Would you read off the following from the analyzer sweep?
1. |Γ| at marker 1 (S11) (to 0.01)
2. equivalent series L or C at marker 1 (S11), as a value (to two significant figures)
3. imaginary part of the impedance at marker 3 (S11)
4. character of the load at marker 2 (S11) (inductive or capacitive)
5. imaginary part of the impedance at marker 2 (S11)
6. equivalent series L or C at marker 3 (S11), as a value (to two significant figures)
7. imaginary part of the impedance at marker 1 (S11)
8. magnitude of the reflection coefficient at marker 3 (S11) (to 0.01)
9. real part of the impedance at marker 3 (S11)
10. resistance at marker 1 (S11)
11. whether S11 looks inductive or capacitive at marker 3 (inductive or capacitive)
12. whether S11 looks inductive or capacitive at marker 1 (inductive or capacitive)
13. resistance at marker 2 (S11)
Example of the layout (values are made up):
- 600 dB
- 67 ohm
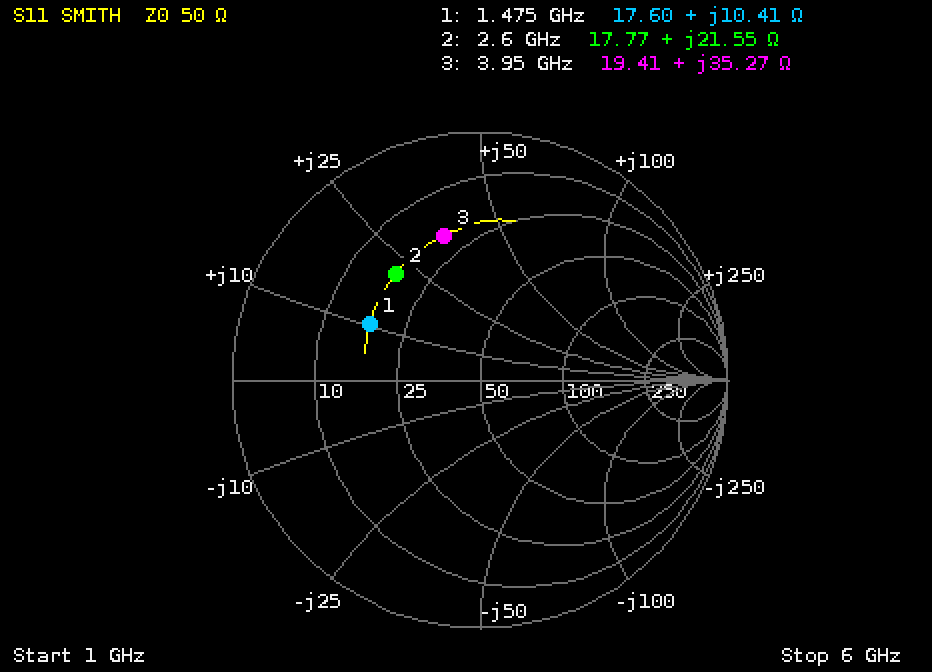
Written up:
- 0.50
- 1.1 nH
- +35.27 Ω
- inductive
- +21.55 Ω
- 1.4 nH
- +10.41 Ω
- 0.60
- 19.41 Ω
- 17.60 Ω
- inductive
- inductive
- 17.77 Ω
